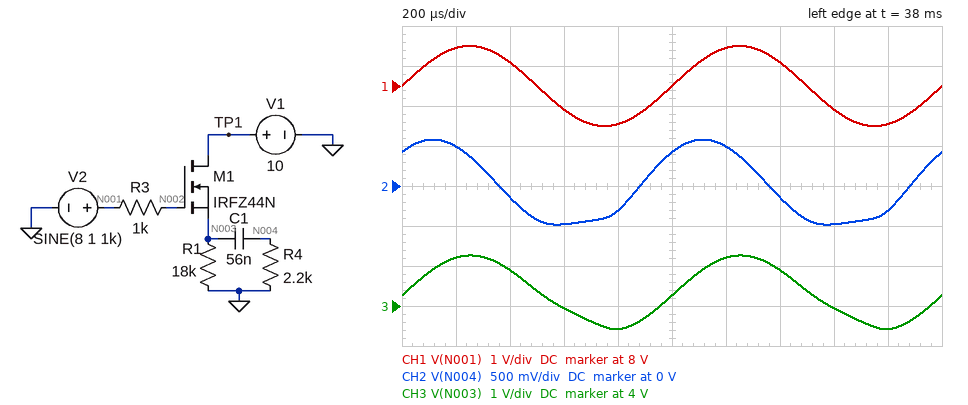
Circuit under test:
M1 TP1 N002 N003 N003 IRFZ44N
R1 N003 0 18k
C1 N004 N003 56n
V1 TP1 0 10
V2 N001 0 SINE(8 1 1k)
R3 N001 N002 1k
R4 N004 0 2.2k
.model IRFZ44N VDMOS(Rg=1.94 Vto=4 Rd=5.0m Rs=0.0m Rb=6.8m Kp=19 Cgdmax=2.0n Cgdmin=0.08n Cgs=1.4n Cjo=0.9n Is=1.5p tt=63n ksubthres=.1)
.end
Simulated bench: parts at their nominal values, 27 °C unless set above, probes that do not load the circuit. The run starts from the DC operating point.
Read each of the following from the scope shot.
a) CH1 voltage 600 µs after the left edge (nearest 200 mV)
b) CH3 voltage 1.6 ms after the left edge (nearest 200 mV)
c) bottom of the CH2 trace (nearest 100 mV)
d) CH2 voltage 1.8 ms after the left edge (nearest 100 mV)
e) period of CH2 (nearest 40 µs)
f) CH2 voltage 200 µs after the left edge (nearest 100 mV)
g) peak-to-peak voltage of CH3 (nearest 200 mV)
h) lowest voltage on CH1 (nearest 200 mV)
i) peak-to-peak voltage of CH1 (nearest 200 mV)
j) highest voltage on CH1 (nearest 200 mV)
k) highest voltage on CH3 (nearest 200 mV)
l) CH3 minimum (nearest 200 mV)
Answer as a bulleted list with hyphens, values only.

- 7.4 V
- 4.0 V
- -500 mV
- -300 mV
- 1.00 ms
- 500 mV
- 1.8 V
- 7.0 V
- 2.0 V
- 9.0 V
- 5.2 V
- 3.4 V
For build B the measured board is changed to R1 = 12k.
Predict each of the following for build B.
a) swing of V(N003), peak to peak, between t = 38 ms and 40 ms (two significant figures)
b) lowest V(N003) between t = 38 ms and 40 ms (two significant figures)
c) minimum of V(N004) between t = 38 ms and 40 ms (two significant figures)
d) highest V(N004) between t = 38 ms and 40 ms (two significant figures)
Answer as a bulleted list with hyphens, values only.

- 1.9 V
- 3.3 V
- -560 mV
- 590 mV
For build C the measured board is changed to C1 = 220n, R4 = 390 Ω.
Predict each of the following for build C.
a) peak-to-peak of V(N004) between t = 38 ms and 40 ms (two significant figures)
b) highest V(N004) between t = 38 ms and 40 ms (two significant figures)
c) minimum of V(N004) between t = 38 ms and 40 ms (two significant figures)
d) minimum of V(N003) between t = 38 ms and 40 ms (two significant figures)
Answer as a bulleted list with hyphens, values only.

- 420 mV
- 310 mV
- -110 mV
- 4.3 V
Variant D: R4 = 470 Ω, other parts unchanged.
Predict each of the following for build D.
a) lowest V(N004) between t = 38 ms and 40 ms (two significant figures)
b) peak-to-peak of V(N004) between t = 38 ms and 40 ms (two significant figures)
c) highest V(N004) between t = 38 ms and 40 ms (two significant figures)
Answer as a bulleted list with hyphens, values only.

- -120 mV
- 280 mV
- 160 mV
